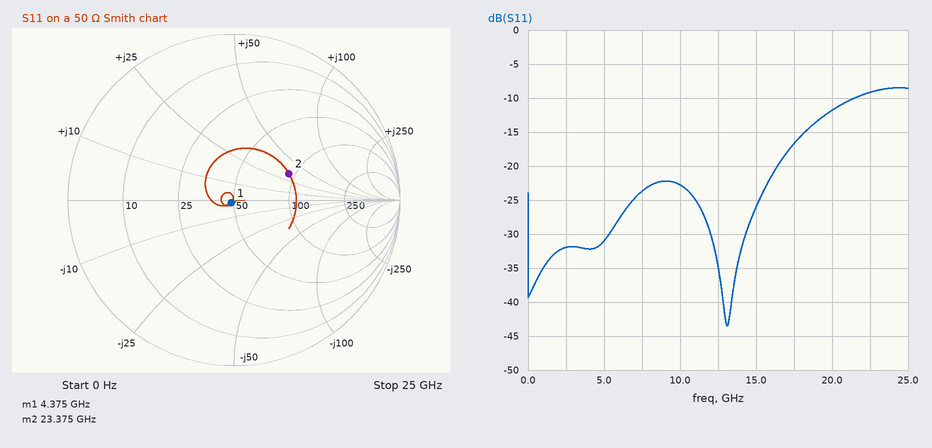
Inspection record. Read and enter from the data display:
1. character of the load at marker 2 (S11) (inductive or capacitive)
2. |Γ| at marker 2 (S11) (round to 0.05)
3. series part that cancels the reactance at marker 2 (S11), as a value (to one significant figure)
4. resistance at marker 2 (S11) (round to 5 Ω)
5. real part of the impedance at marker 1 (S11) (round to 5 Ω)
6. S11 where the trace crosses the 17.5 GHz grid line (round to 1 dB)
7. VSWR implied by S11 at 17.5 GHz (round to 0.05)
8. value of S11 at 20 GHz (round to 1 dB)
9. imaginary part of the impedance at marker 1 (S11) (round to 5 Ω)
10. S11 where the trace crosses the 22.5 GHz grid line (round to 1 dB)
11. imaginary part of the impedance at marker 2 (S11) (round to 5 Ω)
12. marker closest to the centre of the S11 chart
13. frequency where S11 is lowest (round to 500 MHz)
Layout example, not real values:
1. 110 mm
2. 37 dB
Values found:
1. inductive
2. 0.35
3. 200 fF
4. 90 Ω
5. 50 Ω
6. -17 dB
7. 1.35
8. -12 dB
9. 0 Ω
10. -9 dB
11. +35 Ω
12. marker 1
13. 13.0 GHz
